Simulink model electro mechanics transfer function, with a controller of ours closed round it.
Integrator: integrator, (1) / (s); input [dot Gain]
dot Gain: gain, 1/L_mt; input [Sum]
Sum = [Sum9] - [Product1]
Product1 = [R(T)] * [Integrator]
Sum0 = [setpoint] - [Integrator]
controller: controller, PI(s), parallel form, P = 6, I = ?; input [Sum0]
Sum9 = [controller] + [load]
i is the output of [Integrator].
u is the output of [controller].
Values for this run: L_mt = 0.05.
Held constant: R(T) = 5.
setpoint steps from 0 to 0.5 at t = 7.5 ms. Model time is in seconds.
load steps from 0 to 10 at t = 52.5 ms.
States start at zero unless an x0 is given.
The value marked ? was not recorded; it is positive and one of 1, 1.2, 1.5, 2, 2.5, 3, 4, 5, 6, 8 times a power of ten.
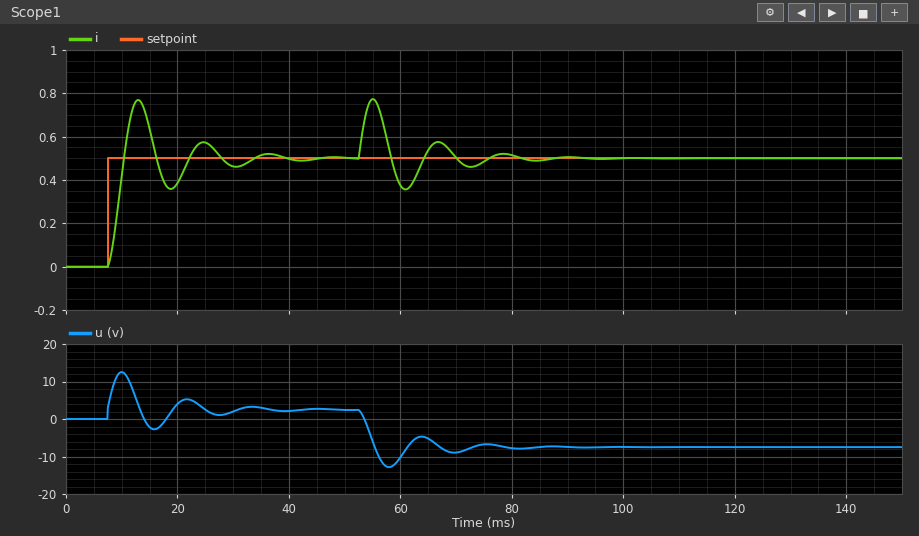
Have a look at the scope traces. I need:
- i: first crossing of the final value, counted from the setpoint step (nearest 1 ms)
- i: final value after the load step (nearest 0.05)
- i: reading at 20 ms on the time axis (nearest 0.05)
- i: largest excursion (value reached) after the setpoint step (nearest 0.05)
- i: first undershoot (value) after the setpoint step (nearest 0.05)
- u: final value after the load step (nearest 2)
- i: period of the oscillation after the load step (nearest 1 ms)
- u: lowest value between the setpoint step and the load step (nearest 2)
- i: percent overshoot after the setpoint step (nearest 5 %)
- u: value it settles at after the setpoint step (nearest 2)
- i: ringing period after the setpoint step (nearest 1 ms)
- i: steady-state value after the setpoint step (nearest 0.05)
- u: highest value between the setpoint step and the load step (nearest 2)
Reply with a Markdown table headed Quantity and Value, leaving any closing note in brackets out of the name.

| Quantity | Value |
|---|---|
| i: first crossing of the final value, counted from the setpoint step | 3 ms |
| i: final value after the load step | 0.50 |
| i: reading at 20 ms on the time axis | 0.40 |
| i: largest excursion (value reached) after the setpoint step | 0.75 |
| i: first undershoot (value) after the setpoint step | 0.35 |
| u: final value after the load step | -8 |
| i: period of the oscillation after the load step | 12 ms |
| u: lowest value between the setpoint step and the load step | -2 |
| i: percent overshoot after the setpoint step | 55 % |
| u: value it settles at after the setpoint step | 2 |
| i: ringing period after the setpoint step | 12 ms |
| i: steady-state value after the setpoint step | 0.50 |
| u: highest value between the setpoint step and the load step | 12 |
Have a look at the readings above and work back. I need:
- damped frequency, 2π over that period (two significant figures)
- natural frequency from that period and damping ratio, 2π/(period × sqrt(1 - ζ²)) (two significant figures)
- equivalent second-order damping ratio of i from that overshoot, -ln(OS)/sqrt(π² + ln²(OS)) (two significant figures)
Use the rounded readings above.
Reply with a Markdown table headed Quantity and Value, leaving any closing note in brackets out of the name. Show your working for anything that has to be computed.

| Quantity | Value |
|---|---|
| damped frequency, 2π over that period | 2π / 12 = 0.52 rad/ms |
| natural frequency from that period and damping ratio, 2π/(period × sqrt(1 - ζ²)) | 2π / (12 × sqrt(1 - 0.19²)) = 0.53 rad/ms |
| equivalent second-order damping ratio of i from that overshoot, -ln(OS)/sqrt(π² + ln²(OS)) | ln(0.55) = -0.598; 0.598 / sqrt(9.870 + 0.357) = 0.19 |
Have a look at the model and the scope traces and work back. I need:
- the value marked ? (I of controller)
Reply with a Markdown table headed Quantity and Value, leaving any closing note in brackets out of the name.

| Quantity | Value |
|---|---|
| the value marked ? | 15000 |
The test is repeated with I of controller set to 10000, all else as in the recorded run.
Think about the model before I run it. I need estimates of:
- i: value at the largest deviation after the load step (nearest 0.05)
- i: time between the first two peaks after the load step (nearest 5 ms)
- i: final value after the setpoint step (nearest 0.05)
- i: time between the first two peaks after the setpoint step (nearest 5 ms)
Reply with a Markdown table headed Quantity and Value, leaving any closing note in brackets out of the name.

| Quantity | Value |
|---|---|
| i: value at the largest deviation after the load step | 0.80 |
| i: time between the first two peaks after the load step | 15 ms |
| i: final value after the setpoint step | 0.50 |
| i: time between the first two peaks after the setpoint step | 15 ms |
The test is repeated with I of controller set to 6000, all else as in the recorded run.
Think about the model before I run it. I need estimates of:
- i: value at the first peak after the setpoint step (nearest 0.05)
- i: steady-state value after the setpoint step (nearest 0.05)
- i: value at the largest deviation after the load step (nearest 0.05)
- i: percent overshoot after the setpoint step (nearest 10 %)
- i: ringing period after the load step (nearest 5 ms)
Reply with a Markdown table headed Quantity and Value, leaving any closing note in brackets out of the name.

| Quantity | Value |
|---|---|
| i: value at the first peak after the setpoint step | 0.70 |
| i: steady-state value after the setpoint step | 0.50 |
| i: value at the largest deviation after the load step | 0.90 |
| i: percent overshoot after the setpoint step | 40 % |
| i: ringing period after the load step | 20 ms |
